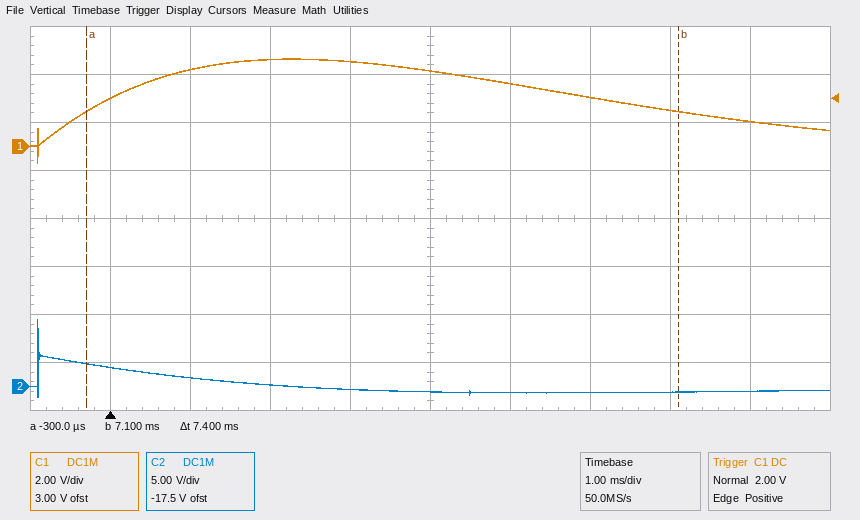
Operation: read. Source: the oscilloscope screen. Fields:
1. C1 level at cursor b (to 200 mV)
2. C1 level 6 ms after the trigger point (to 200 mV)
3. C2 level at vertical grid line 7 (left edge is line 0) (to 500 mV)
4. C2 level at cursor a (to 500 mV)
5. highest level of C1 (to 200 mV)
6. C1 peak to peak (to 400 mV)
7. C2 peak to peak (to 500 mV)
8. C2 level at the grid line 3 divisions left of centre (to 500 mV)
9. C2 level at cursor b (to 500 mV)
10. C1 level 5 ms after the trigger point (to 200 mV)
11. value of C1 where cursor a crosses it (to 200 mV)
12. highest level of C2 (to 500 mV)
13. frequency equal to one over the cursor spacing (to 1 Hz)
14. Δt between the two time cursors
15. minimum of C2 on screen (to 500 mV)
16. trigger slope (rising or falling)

1.4 V
2.0 V
-500 mV
2.5 V
3.6 V
4.4 V
8.0 V
1.0 V
-500 mV
2.6 V
1.4 V
7.0 V
135 Hz
7.4 ms
-1.0 V
rising
